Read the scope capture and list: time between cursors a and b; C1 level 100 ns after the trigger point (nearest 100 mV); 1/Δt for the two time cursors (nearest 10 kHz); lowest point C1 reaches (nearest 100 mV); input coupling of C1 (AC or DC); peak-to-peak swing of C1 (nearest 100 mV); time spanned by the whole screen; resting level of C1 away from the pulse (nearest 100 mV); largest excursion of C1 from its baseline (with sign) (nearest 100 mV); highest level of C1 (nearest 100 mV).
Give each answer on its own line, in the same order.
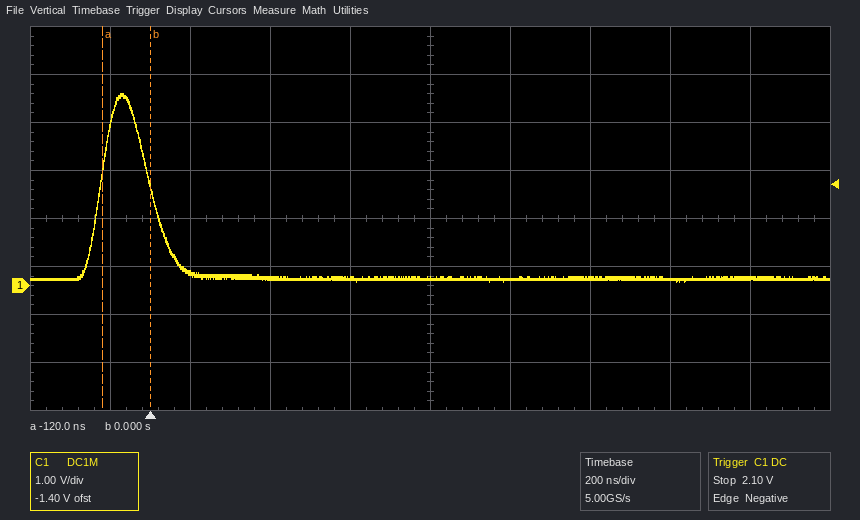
120 ns
300 mV
8.33 MHz
100 mV
DC
3.9 V
2 µs
200 mV
+3.8 V
4.0 V
